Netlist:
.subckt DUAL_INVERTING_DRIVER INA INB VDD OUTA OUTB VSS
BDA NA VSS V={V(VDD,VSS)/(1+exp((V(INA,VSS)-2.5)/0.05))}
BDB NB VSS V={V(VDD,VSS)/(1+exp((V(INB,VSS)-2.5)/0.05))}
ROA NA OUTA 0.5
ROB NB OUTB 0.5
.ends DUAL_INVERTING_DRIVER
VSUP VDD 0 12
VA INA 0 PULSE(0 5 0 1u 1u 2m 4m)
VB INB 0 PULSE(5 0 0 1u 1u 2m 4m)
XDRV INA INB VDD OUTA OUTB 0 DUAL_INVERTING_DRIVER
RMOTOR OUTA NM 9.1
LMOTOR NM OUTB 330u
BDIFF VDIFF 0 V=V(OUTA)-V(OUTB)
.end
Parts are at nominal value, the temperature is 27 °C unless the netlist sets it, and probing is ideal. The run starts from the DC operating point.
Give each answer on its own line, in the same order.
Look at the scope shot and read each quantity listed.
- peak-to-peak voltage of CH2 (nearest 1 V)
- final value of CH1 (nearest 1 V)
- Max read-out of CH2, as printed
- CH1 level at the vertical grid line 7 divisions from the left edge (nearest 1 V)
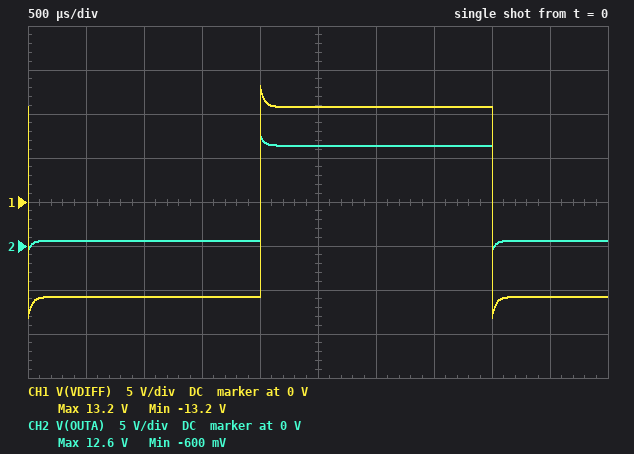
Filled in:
13 V
-11 V
12.6 V
11 V
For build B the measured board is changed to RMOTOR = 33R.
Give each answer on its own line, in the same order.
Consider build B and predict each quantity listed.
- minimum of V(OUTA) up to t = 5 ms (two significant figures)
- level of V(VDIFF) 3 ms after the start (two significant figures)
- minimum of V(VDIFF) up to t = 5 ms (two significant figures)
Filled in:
-170 mV
12 V
-12 V
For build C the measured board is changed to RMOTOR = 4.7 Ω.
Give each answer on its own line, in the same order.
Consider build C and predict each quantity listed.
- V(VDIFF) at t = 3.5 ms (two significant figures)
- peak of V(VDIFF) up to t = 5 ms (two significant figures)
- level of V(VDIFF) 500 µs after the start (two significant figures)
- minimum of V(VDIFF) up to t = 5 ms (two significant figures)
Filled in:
9.9 V
14 V
-9.9 V
-14 V
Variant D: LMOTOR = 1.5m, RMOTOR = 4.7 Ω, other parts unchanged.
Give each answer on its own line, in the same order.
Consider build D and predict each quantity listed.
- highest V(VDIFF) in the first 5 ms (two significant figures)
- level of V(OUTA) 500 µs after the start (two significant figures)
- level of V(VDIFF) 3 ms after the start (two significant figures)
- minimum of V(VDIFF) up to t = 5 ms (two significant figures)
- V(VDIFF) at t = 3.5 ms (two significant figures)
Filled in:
14 V
740 mV
10 V
-14 V
9.9 V
